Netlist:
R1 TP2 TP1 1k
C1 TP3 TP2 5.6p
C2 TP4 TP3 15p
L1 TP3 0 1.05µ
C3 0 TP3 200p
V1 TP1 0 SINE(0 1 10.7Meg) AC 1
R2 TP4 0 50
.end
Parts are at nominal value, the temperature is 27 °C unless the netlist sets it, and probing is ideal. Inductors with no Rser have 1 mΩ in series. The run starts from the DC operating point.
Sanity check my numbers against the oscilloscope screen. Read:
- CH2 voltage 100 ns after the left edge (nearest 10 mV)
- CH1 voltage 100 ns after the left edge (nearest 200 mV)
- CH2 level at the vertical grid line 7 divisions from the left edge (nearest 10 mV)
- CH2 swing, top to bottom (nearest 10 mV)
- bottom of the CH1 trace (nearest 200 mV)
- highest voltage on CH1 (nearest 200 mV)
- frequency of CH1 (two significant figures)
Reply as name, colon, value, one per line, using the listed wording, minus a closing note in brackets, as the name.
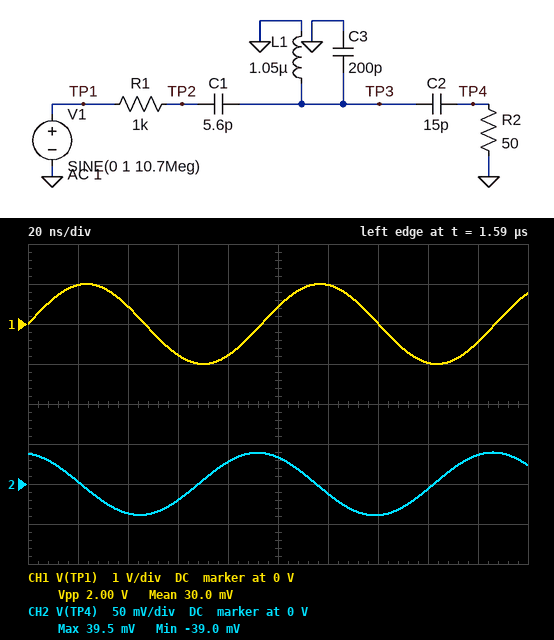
CH2 voltage 100 ns after the left edge: 30 mV
CH1 voltage 100 ns after the left edge: 400 mV
CH2 level at the vertical grid line 7 divisions from the left edge: -40 mV
CH2 swing, top to bottom: 80 mV
bottom of the CH1 trace: -1.0 V
highest voltage on CH1: 1.0 V
frequency of CH1: 11 MHz
